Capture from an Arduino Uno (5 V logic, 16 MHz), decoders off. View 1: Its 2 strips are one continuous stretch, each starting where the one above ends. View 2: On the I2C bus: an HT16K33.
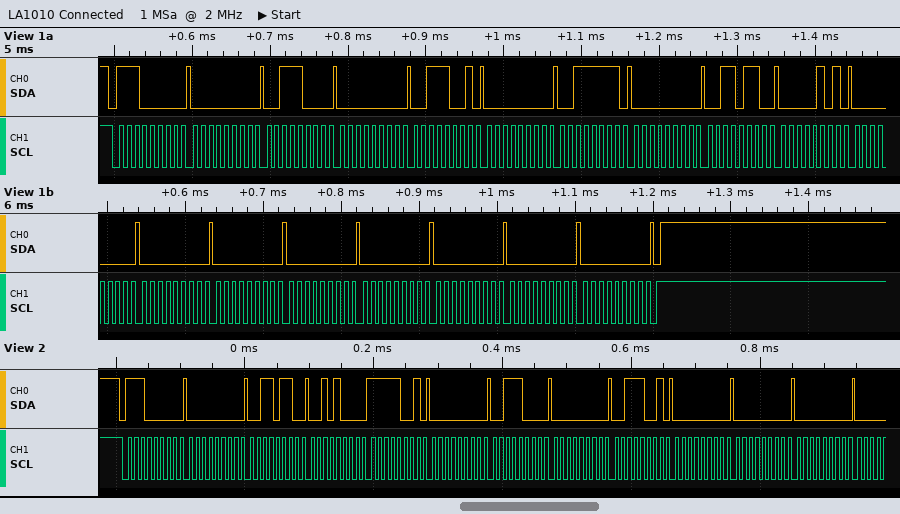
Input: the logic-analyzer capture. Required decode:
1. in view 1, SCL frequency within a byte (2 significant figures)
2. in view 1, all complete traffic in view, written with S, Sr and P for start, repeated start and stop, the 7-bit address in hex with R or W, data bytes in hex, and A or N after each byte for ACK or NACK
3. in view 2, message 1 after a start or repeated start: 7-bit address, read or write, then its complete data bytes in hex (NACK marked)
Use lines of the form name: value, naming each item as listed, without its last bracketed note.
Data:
in view 1, SCL frequency within a byte: 100 kHz
in view 1, all complete traffic in view, written with S, Sr and P for start, repeated start and stop, the 7-bit address in hex with R or W, data bytes in hex, and A or N after each byte for ACK or NACK: S 70W A 00 A 38 A 00 A 39 A 00 A 3F A 00 A 36 A 05 A 00 A 00 A 00 A 00 A 00 A 00 A 00 A 00 A P
in view 2, message 1 after a start or repeated start: 7-bit address, read or write, then its complete data bytes in hex: 0x70 write: 00 36 28 F9 00 38 00 39 00 00 00
